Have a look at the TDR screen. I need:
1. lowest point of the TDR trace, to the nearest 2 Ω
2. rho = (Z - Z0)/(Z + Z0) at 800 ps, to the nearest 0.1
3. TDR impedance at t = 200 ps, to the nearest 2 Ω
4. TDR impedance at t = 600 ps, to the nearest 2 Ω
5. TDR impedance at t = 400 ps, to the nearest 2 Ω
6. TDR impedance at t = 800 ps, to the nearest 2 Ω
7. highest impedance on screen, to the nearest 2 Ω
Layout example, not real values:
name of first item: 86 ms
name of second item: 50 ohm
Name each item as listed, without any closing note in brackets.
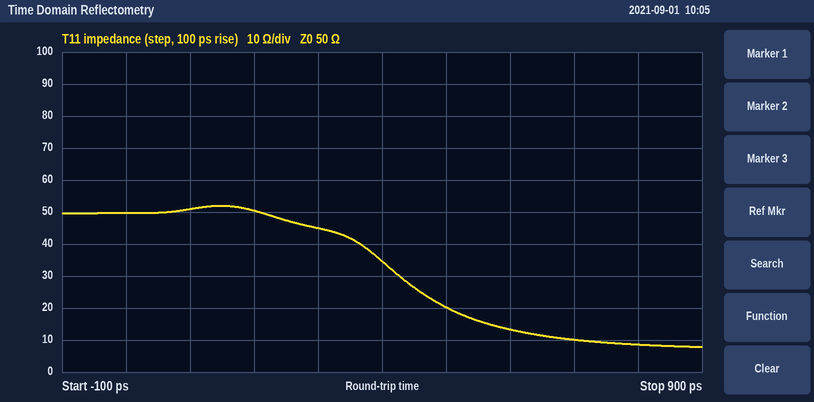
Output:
lowest point of the TDR trace, to the nearest 2 Ω: 8 Ω
rho = (Z - Z0)/(Z + Z0) at 800 ps, to the nearest 0.1: -0.7
TDR impedance at t = 200 ps, to the nearest 2 Ω: 50 Ω
TDR impedance at t = 600 ps, to the nearest 2 Ω: 14 Ω
TDR impedance at t = 400 ps, to the nearest 2 Ω: 34 Ω
TDR impedance at t = 800 ps, to the nearest 2 Ω: 8 Ω
highest impedance on screen, to the nearest 2 Ω: 52 Ω
